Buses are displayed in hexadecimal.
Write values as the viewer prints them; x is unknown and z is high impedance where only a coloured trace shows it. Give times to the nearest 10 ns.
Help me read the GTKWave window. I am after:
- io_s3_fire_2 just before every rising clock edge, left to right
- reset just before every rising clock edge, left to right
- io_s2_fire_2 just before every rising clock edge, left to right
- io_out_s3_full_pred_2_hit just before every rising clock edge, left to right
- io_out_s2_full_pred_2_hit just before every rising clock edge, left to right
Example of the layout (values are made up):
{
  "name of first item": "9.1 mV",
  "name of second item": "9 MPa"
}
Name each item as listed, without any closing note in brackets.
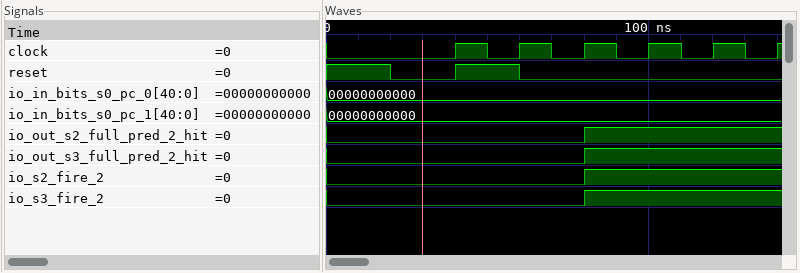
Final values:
{
  "io_s3_fire_2 just before every rising clock edge, left to right": "0 0 0 1 1 1",
  "reset just before every rising clock edge, left to right": "0 1 0 0 0 0",
  "io_s2_fire_2 just before every rising clock edge, left to right": "0 0 0 1 1 1",
  "io_out_s3_full_pred_2_hit just before every rising clock edge, left to right": "0 0 0 1 1 1",
  "io_out_s2_full_pred_2_hit just before every rising clock edge, left to right": "0 0 0 1 1 1"
}
